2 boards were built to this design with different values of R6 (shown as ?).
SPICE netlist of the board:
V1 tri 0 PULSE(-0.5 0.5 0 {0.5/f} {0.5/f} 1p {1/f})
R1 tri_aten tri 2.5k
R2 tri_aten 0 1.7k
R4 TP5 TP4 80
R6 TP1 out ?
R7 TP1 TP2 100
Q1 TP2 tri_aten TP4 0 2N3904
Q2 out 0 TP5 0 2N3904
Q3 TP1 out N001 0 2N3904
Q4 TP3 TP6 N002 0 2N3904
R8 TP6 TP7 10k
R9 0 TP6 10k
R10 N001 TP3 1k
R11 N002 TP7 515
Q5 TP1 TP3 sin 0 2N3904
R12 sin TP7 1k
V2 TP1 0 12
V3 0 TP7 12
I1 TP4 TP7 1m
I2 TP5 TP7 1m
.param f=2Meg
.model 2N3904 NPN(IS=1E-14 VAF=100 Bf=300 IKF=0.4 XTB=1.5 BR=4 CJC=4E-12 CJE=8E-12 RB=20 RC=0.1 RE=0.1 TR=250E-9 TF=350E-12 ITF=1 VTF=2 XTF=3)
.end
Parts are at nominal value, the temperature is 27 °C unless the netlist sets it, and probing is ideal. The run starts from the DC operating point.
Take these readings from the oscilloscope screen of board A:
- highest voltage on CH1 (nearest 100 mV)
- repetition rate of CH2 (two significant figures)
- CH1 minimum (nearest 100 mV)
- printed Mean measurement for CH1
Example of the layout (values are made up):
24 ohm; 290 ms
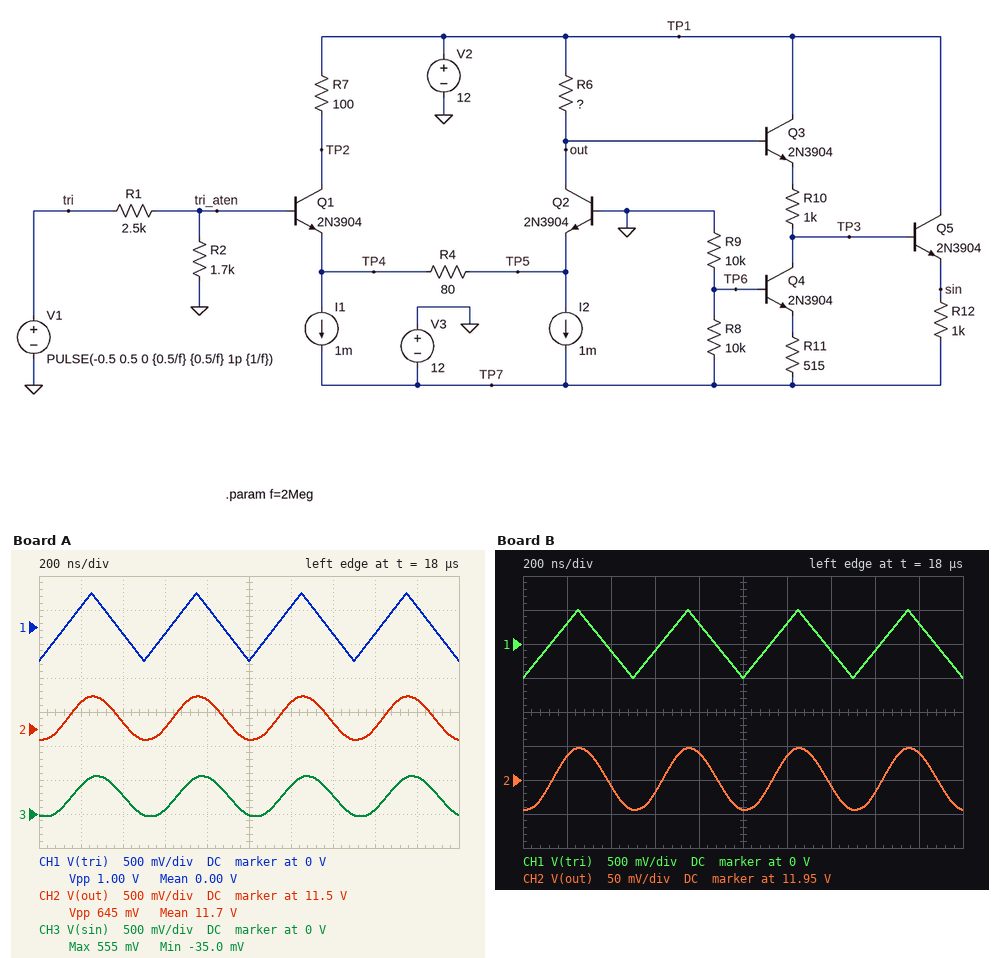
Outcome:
500 mV; 2.0 MHz; -500 mV; 0.00 V
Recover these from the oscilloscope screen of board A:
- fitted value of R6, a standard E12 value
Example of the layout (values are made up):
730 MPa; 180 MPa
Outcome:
330 Ω
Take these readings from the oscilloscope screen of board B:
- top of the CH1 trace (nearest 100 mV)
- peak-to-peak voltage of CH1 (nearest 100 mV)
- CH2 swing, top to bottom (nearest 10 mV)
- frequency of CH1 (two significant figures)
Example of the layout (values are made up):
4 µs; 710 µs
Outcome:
500 mV; 1.0 V; 90 mV; 2.0 MHz
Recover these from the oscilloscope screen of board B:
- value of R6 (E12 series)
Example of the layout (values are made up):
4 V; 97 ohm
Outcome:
47 Ω
